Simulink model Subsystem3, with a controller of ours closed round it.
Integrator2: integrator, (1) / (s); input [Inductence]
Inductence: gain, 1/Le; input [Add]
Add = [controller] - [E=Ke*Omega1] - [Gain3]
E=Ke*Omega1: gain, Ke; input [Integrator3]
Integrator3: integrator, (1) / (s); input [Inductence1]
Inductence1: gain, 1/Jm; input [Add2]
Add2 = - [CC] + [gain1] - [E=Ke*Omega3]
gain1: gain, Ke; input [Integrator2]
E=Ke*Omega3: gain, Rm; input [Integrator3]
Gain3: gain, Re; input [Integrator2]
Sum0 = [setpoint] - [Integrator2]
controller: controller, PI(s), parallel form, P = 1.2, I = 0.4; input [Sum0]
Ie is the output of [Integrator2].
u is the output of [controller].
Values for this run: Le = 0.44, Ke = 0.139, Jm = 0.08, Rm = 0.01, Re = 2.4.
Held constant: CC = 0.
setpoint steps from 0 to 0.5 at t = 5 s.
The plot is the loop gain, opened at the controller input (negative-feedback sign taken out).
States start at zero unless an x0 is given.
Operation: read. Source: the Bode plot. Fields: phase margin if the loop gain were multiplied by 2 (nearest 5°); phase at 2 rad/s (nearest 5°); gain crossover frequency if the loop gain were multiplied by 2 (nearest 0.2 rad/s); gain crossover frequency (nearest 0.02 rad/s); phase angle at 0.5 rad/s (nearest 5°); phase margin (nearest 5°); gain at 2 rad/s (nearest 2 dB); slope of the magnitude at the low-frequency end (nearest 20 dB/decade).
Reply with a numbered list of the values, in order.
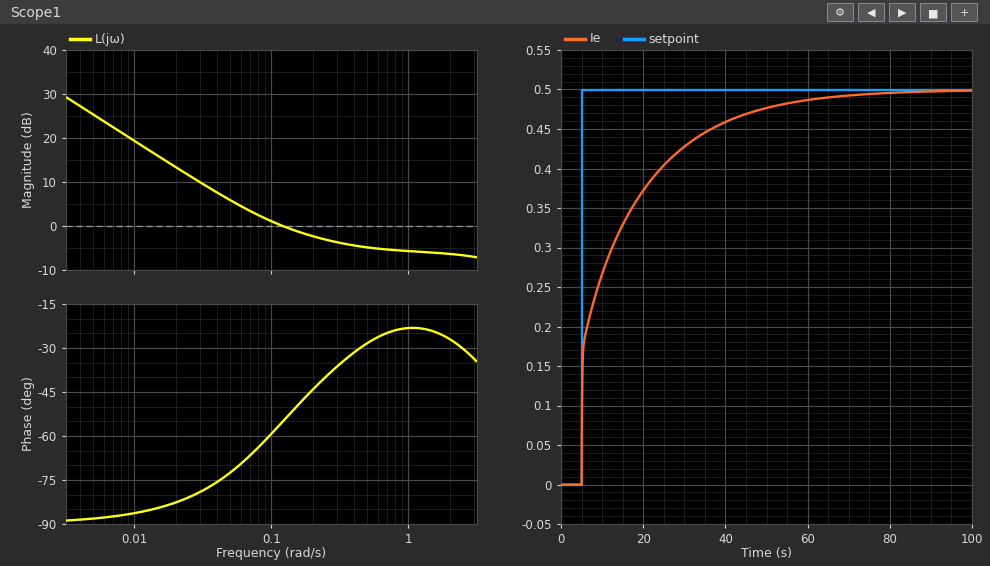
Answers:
1. 155°
2. -25°
3. 1.4 rad/s
4. 0.12 rad/s
5. -30°
6. 125°
7. -6 dB
8. -20 dB/decade
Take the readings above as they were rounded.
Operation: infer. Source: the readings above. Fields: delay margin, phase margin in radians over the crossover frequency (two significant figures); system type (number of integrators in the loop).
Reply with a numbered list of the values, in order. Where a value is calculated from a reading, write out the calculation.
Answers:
1. 125 × π / 180 / 0.12 = 18 s
2. 1
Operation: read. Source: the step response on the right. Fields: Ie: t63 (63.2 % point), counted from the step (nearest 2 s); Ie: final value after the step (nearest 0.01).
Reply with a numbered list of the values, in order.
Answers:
1. 8 s
2. 0.50
